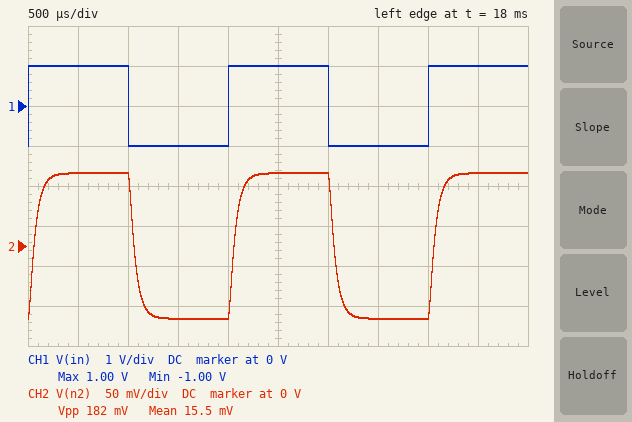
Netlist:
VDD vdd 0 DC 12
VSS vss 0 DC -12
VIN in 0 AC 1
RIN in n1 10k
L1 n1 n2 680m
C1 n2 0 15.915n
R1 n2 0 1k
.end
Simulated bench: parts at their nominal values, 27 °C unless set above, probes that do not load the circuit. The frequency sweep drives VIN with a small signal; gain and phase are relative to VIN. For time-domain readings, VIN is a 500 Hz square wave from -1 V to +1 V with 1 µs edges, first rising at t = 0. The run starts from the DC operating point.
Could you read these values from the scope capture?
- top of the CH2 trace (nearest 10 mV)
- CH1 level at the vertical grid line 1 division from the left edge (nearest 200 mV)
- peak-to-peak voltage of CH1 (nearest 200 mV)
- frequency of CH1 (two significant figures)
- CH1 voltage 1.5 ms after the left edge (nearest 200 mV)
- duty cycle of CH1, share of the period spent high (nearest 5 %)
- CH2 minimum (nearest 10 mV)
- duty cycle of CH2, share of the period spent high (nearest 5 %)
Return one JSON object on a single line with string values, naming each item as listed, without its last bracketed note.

{"top of the CH2 trace": "90 mV", "CH1 level at the vertical grid line 1 division from the left edge": "1.0 V", "peak-to-peak voltage of CH1": "2.0 V", "frequency of CH1": "500 Hz", "CH1 voltage 1.5 ms after the left edge": "-1.0 V", "duty cycle of CH1, share of the period spent high": "50 %", "CH2 minimum": "-90 mV", "duty cycle of CH2, share of the period spent high": "50 %"}
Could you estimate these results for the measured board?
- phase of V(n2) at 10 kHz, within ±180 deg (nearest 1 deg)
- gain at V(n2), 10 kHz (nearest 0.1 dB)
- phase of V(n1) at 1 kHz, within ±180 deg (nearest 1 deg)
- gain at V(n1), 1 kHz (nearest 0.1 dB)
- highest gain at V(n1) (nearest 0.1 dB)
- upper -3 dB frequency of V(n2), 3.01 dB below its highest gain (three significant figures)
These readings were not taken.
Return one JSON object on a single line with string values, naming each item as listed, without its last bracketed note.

{"phase of V(n2) at 10 kHz, within ±180 deg": "-121 deg", "gain at V(n2), 10 kHz": "-35.8 dB", "phase of V(n1) at 1 kHz, within ±180 deg": "56 deg", "gain at V(n1), 1 kHz": "-8.8 dB", "highest gain at V(n1)": "0 dB", "upper -3 dB frequency of V(n2), 3.01 dB below its highest gain": "2.49 kHz"}
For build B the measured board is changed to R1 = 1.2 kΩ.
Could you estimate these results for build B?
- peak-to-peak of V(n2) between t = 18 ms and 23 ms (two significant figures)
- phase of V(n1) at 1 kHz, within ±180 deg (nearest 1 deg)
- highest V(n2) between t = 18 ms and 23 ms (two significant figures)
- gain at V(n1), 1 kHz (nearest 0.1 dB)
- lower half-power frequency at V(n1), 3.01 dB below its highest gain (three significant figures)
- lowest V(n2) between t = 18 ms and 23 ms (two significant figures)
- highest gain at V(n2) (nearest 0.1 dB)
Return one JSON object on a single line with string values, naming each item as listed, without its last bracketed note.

{"peak-to-peak of V(n2) between t = 18 ms and 23 ms": "210 mV", "phase of V(n1) at 1 kHz, within ±180 deg": "54 deg", "highest V(n2) between t = 18 ms and 23 ms": "110 mV", "gain at V(n1), 1 kHz": "-8.9 dB", "lower half-power frequency at V(n1), 3.01 dB below its highest gain": "2.65 kHz", "lowest V(n2) between t = 18 ms and 23 ms": "-110 mV", "highest gain at V(n2)": "-19.4 dB"}
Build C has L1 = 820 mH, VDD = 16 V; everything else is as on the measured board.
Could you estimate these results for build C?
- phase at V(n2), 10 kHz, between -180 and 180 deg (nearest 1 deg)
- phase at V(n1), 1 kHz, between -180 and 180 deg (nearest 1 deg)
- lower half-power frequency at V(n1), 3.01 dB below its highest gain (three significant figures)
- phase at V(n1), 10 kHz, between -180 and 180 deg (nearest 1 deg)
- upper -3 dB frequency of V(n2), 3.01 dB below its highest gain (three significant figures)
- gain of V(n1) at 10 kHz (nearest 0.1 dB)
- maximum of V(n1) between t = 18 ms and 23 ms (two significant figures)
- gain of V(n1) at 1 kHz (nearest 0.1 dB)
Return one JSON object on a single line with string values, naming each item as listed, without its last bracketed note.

{"phase at V(n2), 10 kHz, between -180 and 180 deg": "-123 deg", "phase at V(n1), 1 kHz, between -180 and 180 deg": "54 deg", "lower half-power frequency at V(n1), 3.01 dB below its highest gain": "2.15 kHz", "phase at V(n1), 10 kHz, between -180 and 180 deg": "11 deg", "upper -3 dB frequency of V(n2), 3.01 dB below its highest gain": "2.09 kHz", "gain of V(n1) at 10 kHz": "-0.2 dB", "maximum of V(n1) between t = 18 ms and 23 ms": "1.9 V", "gain of V(n1) at 1 kHz": "-7.4 dB"}
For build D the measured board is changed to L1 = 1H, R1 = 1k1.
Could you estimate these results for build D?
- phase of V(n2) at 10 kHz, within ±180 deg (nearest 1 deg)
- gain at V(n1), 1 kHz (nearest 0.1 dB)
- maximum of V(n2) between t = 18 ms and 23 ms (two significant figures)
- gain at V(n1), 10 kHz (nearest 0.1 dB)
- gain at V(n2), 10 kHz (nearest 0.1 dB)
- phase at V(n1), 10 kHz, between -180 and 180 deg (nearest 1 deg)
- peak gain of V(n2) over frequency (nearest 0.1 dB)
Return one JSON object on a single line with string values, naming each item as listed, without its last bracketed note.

{"phase of V(n2) at 10 kHz, within ±180 deg": "-128 deg", "gain at V(n1), 1 kHz": "-6.1 dB", "maximum of V(n2) between t = 18 ms and 23 ms": "99 mV", "gain at V(n1), 10 kHz": "-0.1 dB", "gain at V(n2), 10 kHz": "-38.6 dB", "phase at V(n1), 10 kHz, between -180 and 180 deg": "9 deg", "peak gain of V(n2) over frequency": "-20.1 dB"}
